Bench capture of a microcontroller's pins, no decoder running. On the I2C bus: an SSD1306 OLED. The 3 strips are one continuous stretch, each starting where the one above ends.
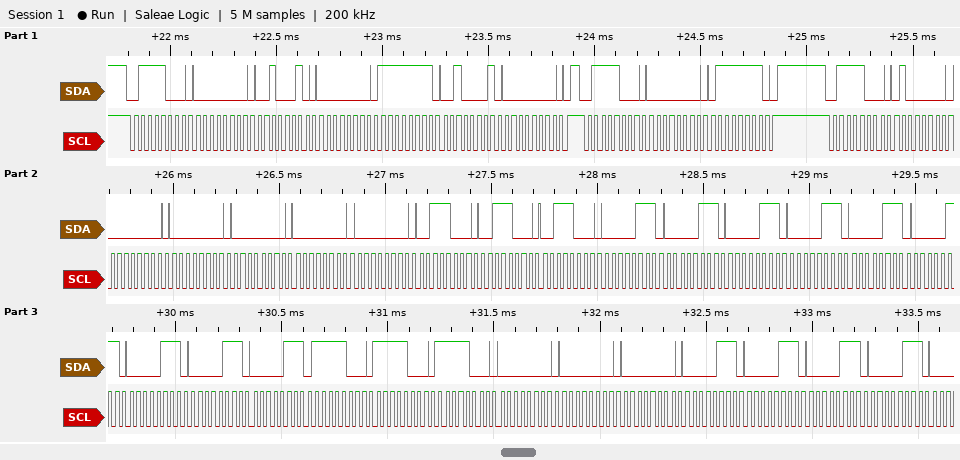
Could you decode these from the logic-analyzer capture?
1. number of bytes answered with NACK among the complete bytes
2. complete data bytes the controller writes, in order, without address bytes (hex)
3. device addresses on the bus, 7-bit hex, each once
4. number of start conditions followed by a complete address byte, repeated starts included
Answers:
0
00 22 00 FF 21 00 00 7F 40 00 00 00 00 00 38 38 38 07 07 07 07 07 07 07 07 07 F8 F8 F8 00 00 00 07 07 07 07
0x3C
3
